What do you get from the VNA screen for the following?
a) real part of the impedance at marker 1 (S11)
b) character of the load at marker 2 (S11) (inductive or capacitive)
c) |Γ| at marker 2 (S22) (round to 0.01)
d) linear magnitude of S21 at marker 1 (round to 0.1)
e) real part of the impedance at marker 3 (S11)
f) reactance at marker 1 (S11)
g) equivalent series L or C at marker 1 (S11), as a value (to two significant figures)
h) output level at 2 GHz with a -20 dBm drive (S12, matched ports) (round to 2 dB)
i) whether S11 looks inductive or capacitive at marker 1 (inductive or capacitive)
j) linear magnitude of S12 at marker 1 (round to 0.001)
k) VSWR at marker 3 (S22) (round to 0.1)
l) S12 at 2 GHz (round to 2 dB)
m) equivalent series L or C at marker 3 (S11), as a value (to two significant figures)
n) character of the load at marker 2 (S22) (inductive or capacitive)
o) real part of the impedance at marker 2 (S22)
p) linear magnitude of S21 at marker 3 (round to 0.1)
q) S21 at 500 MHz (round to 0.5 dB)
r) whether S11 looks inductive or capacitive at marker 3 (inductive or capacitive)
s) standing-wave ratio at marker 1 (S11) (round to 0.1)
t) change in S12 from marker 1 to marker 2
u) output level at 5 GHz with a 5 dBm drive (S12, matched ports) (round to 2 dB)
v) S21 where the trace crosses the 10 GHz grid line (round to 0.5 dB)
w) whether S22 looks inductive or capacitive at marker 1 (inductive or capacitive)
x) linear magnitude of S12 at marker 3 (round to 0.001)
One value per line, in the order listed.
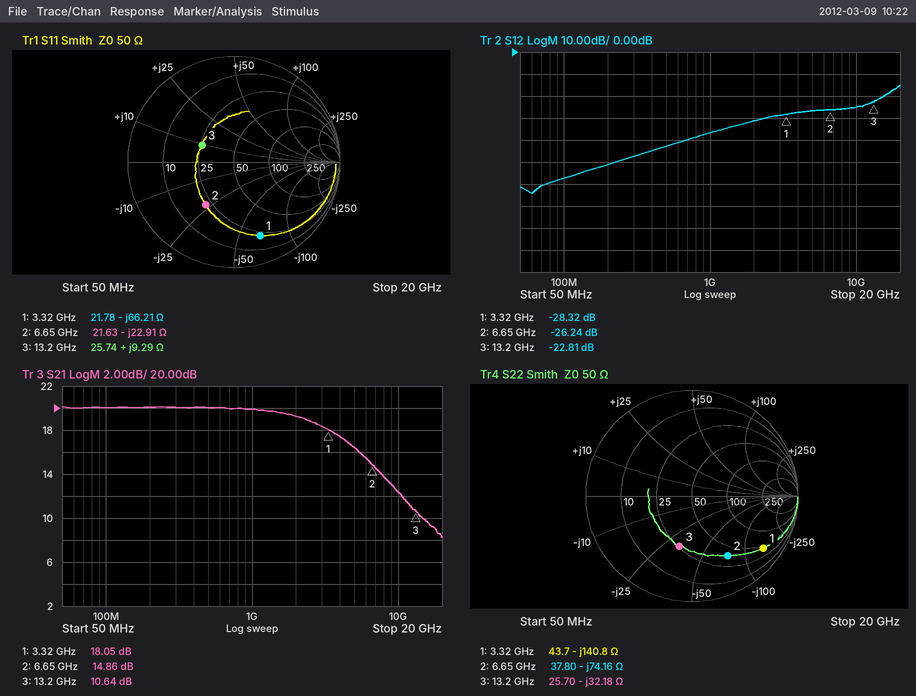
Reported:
21.78 Ω
capacitive
0.65
8.0
25.74 Ω
-66.21 Ω
720 fF
-52 dBm
capacitive
0.038
2.9
-32 dB
110 pH
capacitive
37.80 Ω
3.4
20.0 dB
inductive
6.6
2.08 dB
-22 dBm
12.5 dB
capacitive
0.072
